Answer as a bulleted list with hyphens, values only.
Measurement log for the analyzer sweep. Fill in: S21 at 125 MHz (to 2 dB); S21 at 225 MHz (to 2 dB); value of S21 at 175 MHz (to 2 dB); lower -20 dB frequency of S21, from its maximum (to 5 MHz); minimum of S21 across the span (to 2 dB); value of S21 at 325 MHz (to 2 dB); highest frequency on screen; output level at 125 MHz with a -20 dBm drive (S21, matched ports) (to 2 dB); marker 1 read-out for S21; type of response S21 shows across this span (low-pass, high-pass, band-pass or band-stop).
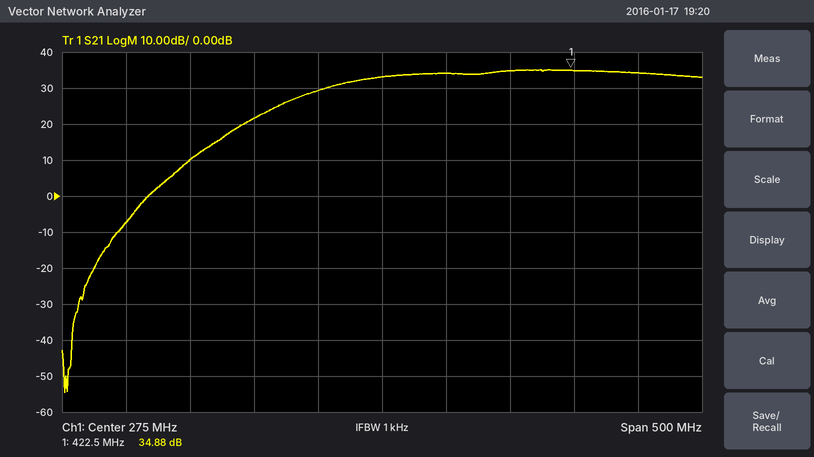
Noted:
- 10 dB
- 30 dB
- 22 dB
- 145 MHz
- -54 dB
- 34 dB
- 525 MHz
- -10 dBm
- 34.88 dB
- high-pass
